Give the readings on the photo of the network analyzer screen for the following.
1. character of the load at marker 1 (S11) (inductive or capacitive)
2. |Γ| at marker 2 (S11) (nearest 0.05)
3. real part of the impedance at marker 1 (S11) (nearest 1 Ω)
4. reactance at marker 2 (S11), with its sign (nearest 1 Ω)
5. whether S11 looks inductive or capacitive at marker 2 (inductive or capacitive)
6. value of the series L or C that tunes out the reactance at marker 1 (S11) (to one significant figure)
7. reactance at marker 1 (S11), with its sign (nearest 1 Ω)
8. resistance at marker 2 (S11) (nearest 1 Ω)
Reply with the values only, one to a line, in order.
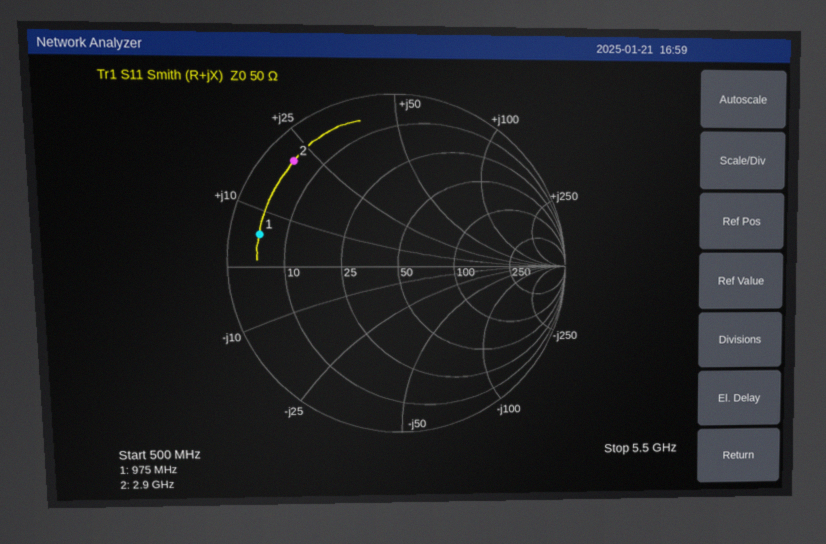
inductive
0.85
5 Ω
+21 Ω
inductive
30 pF
+6 Ω
5 Ω
